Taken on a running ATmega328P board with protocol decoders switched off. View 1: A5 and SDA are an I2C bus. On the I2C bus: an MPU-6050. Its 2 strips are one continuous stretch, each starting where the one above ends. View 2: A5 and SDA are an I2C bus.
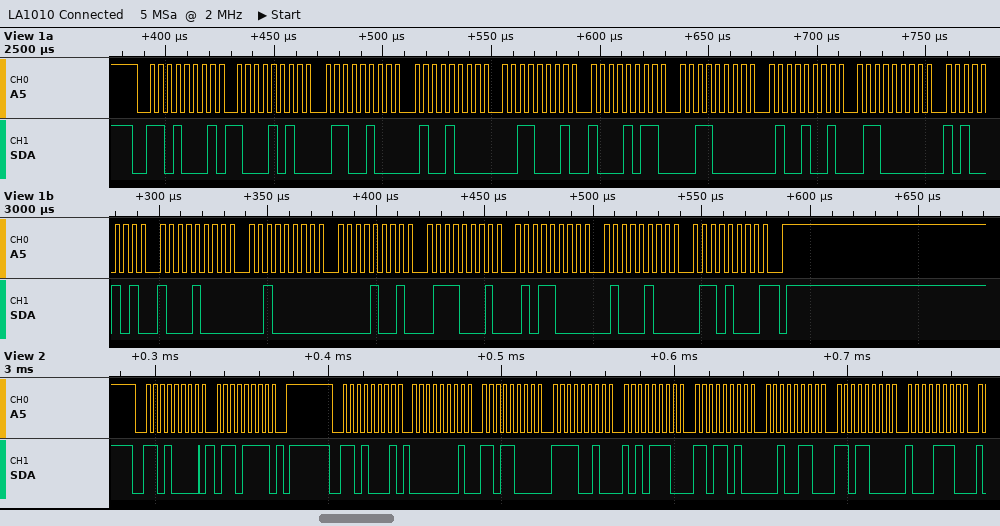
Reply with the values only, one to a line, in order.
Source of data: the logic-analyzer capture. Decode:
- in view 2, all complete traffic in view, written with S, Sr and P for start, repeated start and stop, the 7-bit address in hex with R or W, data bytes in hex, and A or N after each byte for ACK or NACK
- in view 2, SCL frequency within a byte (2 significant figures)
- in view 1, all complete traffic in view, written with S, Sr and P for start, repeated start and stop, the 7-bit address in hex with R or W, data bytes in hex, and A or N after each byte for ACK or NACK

S 68W A 6F A P S 68R A 01 A D8 A F2 A AE A DA A 26 A D8 A 8E A
250 kHz
S 68R A 8A A 64 A 48 A 31 A 8B A 30 A 49 A 60 A A5 A 88 A 20 A 09 A 71 A 58 A 44 A 68 N P
